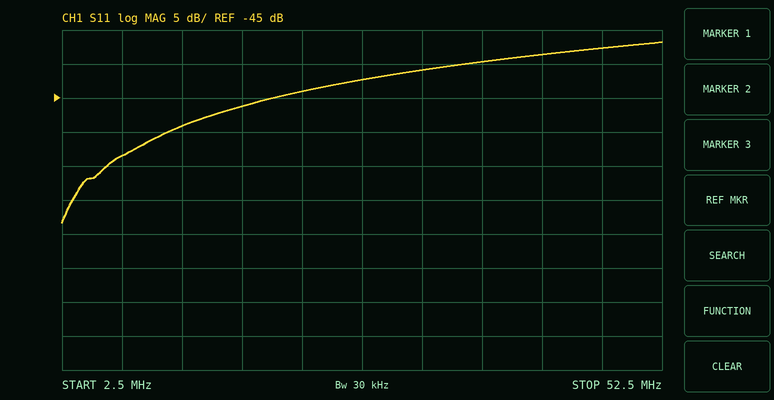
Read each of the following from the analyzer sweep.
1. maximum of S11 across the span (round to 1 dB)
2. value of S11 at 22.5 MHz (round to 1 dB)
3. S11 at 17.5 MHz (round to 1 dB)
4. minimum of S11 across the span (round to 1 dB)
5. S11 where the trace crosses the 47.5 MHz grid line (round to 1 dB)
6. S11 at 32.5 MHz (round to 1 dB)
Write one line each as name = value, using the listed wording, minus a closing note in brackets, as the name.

maximum of S11 across the span = -37 dB
value of S11 at 22.5 MHz = -44 dB
S11 at 17.5 MHz = -46 dB
minimum of S11 across the span = -63 dB
S11 where the trace crosses the 47.5 MHz grid line = -38 dB
S11 at 32.5 MHz = -41 dB
